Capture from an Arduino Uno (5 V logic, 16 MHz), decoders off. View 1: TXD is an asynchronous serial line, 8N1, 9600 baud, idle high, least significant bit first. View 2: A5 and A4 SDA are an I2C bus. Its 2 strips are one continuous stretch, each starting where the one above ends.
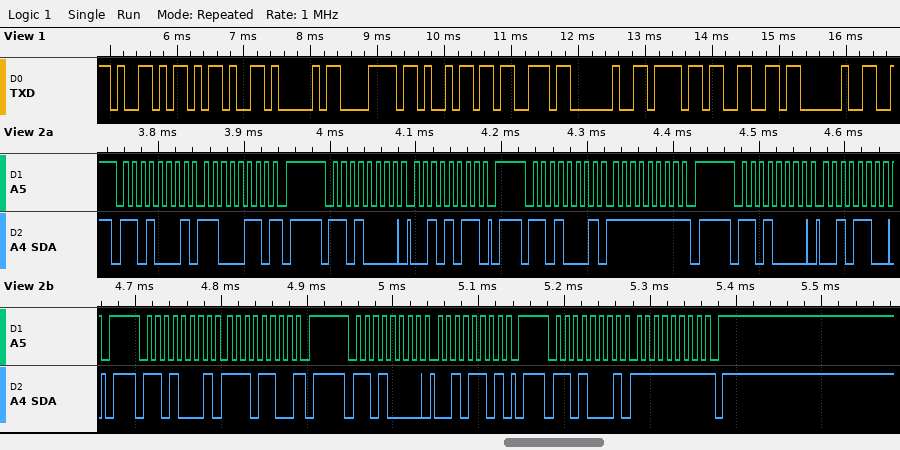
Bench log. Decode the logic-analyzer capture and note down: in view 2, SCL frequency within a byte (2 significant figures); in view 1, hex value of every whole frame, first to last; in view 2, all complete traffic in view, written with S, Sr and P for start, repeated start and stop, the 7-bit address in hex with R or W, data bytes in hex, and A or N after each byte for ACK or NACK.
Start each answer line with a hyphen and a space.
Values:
- 100 kHz
- 0x59 0x2D 0x41 0x78 0x69 0x73 0x20 0x6F 0x66 0x20
- S 68R A C6 N P S 68W A 2B A P S 68R A FF N P S 68W A 2C A P S 68R A EC N P S 68W A 2D A P S 68R A FF N P
